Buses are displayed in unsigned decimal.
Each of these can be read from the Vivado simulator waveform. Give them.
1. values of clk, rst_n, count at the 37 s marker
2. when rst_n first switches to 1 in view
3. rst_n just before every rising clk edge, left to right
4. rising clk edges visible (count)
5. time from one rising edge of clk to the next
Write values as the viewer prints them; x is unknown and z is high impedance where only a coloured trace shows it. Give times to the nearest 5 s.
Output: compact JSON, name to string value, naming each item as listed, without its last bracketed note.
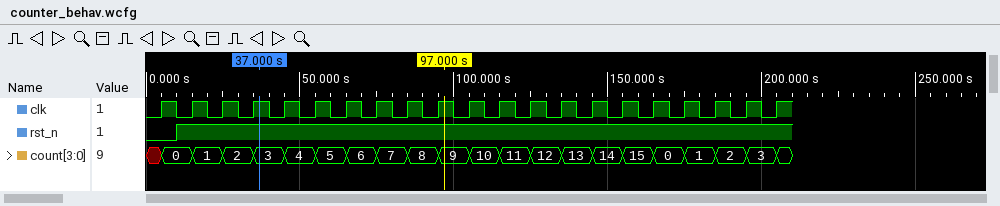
{"values of clk, rst_n, count at the 37 s marker": "clk=1, rst_n=1, count=3", "when rst_n first switches to 1 in view": "10 s", "rst_n just before every rising clk edge, left to right": "0 1 1 1 1 1 1 1 1 1 1 1 1 1 1 1 1 1 1 1 1", "rising clk edges visible": "21", "time from one rising edge of clk to the next": "10 s"}
